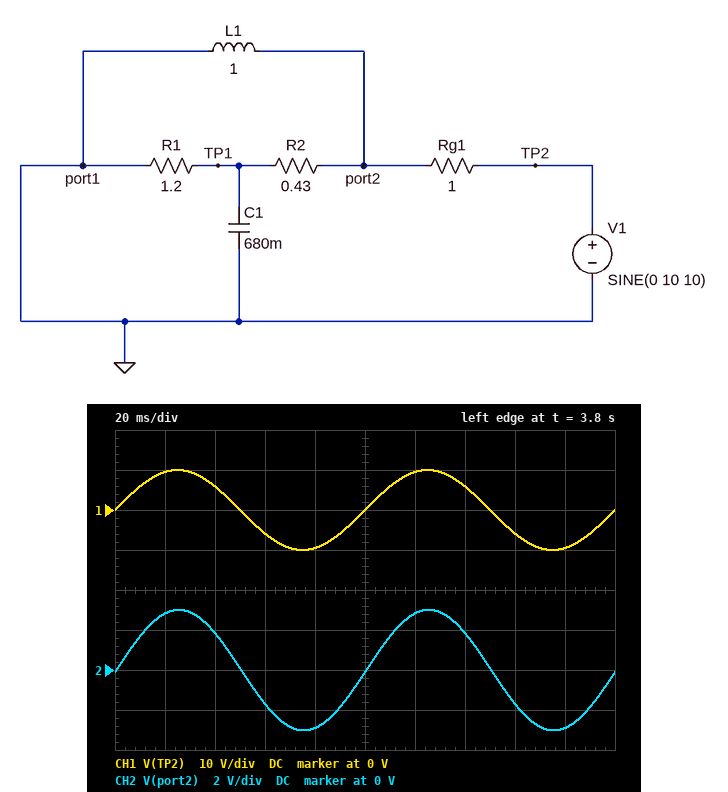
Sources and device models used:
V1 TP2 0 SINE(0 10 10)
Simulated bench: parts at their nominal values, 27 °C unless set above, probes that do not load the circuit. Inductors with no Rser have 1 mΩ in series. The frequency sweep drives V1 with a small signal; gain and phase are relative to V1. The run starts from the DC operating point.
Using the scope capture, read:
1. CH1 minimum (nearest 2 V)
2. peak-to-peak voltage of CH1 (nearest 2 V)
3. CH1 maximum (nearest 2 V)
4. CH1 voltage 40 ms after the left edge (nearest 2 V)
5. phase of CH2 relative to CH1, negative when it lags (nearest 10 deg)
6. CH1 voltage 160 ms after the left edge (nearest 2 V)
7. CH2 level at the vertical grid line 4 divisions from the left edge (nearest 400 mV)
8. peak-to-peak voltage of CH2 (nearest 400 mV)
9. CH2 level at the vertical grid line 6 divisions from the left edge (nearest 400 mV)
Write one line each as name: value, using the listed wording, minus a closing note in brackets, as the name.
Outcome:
CH1 minimum: -10 V
peak-to-peak voltage of CH1: 20 V
CH1 maximum: 10 V
CH1 voltage 40 ms after the left edge: 6 V
phase of CH2 relative to CH1, negative when it lags: 0 deg
CH1 voltage 160 ms after the left edge: -6 V
CH2 level at the vertical grid line 4 divisions from the left edge: -2.8 V
peak-to-peak voltage of CH2: 6.0 V
CH2 level at the vertical grid line 6 divisions from the left edge: 2.8 V
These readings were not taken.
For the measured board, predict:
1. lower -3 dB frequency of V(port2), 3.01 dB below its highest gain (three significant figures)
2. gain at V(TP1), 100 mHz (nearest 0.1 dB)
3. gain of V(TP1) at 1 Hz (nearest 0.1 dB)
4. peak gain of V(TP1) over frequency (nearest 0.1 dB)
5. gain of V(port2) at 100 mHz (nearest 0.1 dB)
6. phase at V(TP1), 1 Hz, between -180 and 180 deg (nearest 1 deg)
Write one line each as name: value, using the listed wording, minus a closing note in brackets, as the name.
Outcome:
lower -3 dB frequency of V(port2), 3.01 dB below its highest gain: 77.0 mHz
gain at V(TP1), 100 mHz: -9.3 dB
gain of V(TP1) at 1 Hz: -16.1 dB
peak gain of V(TP1) over frequency: -7.9 dB
gain of V(port2) at 100 mHz: -6.6 dB
phase at V(TP1), 1 Hz, between -180 and 180 deg: -67 deg
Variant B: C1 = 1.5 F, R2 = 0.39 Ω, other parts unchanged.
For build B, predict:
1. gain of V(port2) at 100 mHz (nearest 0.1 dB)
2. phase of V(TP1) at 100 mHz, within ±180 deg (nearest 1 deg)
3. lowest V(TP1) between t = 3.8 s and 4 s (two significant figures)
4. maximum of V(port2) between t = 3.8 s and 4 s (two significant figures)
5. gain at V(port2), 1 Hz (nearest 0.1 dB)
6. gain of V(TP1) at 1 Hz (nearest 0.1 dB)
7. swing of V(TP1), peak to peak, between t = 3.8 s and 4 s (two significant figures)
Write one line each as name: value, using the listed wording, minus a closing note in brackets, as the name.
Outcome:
gain of V(port2) at 100 mHz: -6.4 dB
phase of V(TP1) at 100 mHz, within ±180 deg: 16 deg
lowest V(TP1) between t = 3.8 s and 4 s: -86 mV
maximum of V(port2) between t = 3.8 s and 4 s: 2.8 V
gain at V(port2), 1 Hz: -10.6 dB
gain of V(TP1) at 1 Hz: -22.4 dB
swing of V(TP1), peak to peak, between t = 3.8 s and 4 s: 150 mV
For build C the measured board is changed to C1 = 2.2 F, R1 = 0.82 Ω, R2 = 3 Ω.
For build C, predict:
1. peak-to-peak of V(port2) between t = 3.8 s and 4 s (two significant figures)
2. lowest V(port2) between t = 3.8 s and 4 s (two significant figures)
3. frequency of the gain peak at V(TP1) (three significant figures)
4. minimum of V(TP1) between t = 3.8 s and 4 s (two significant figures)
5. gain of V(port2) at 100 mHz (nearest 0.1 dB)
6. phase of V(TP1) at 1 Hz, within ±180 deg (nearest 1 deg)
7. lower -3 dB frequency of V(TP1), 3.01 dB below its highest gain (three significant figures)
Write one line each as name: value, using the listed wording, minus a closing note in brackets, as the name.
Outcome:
peak-to-peak of V(port2) between t = 3.8 s and 4 s: 15 V
lowest V(port2) between t = 3.8 s and 4 s: -7.5 V
frequency of the gain peak at V(TP1): 116 mHz
minimum of V(TP1) between t = 3.8 s and 4 s: -20 mV
gain of V(port2) at 100 mHz: -6.1 dB
phase of V(TP1) at 1 Hz, within ±180 deg: -77 deg
lower -3 dB frequency of V(TP1), 3.01 dB below its highest gain: 48.9 mHz
